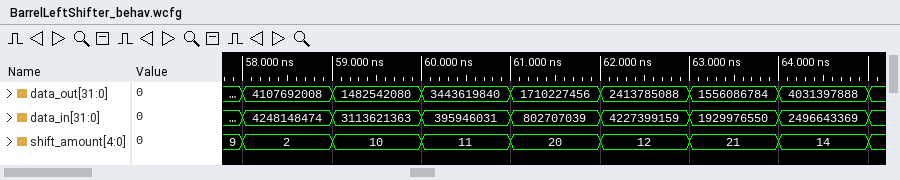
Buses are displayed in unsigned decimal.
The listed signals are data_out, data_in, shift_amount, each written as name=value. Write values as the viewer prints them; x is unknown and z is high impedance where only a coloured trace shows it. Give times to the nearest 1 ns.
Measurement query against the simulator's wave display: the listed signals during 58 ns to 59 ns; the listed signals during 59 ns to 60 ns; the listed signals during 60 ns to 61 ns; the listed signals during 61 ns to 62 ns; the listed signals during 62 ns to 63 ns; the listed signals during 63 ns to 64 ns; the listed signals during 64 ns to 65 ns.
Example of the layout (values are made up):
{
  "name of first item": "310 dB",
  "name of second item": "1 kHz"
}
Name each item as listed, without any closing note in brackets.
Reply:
{
  "the listed signals during 58 ns to 59 ns": "data_out=4107692008, data_in=4248148474, shift_amount=2",
  "the listed signals during 59 ns to 60 ns": "data_out=1482542080, data_in=3113621363, shift_amount=10",
  "the listed signals during 60 ns to 61 ns": "data_out=3443619840, data_in=395946031, shift_amount=11",
  "the listed signals during 61 ns to 62 ns": "data_out=1710227456, data_in=802707039, shift_amount=20",
  "the listed signals during 62 ns to 63 ns": "data_out=2413785088, data_in=4227399159, shift_amount=12",
  "the listed signals during 63 ns to 64 ns": "data_out=1556086784, data_in=1929976550, shift_amount=21",
  "the listed signals during 64 ns to 65 ns": "data_out=4031397888, data_in=2496643369, shift_amount=14"
}
